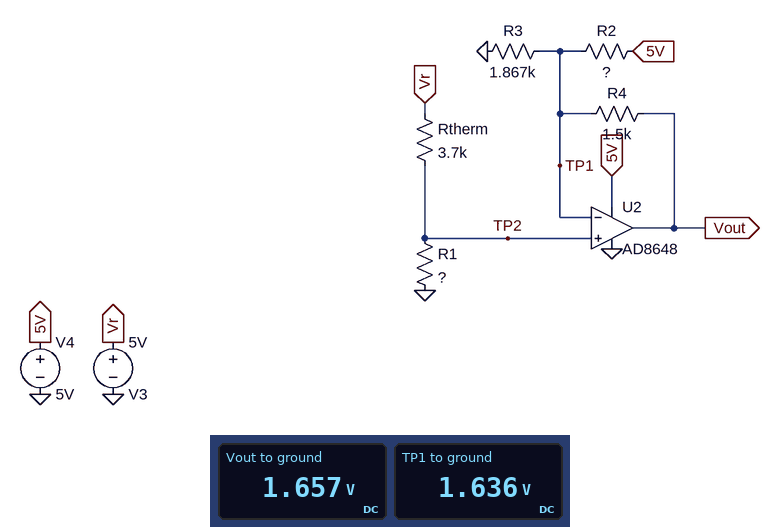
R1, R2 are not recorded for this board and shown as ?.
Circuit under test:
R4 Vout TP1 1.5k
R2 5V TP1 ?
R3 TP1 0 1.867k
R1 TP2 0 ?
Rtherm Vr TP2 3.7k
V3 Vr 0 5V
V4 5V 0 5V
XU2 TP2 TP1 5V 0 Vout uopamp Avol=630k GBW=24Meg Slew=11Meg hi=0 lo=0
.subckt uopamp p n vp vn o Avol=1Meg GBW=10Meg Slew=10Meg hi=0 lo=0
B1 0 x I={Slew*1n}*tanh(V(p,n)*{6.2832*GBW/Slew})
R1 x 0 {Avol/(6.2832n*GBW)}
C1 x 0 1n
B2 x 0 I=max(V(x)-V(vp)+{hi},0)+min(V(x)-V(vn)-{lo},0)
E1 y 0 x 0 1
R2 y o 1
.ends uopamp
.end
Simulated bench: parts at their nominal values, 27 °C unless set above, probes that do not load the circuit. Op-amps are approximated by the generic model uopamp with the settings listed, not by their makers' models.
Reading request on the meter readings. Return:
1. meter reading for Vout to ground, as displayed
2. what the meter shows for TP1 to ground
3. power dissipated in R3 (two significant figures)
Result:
1.657 V
1.636 V
1.4 mW
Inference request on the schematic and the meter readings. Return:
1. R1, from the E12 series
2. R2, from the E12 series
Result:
1.8 kΩ
3.9 kΩ
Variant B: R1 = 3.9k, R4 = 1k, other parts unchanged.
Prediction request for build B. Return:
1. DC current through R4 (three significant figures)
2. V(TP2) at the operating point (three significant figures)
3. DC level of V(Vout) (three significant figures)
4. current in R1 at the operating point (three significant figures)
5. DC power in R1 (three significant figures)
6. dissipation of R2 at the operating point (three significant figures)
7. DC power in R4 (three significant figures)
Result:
750 µA
2.57 V
3.32 V
658 µA
1.69 mW
1.52 mW
563 µW
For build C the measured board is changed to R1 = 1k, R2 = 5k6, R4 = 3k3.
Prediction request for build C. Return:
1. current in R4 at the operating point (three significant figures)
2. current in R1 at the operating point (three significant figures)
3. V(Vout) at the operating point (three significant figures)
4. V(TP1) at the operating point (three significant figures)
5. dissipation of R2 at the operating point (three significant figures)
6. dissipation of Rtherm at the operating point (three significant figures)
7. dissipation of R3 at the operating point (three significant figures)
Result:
133 µA
1.06 mA
625 mV
1.06 V
2.77 mW
4.19 mW
606 µW
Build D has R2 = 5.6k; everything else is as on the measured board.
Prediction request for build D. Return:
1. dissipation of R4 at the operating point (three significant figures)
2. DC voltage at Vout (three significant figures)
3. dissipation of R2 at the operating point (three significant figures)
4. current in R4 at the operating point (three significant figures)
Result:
114 µW
2.05 V
2.02 mW
276 µA
